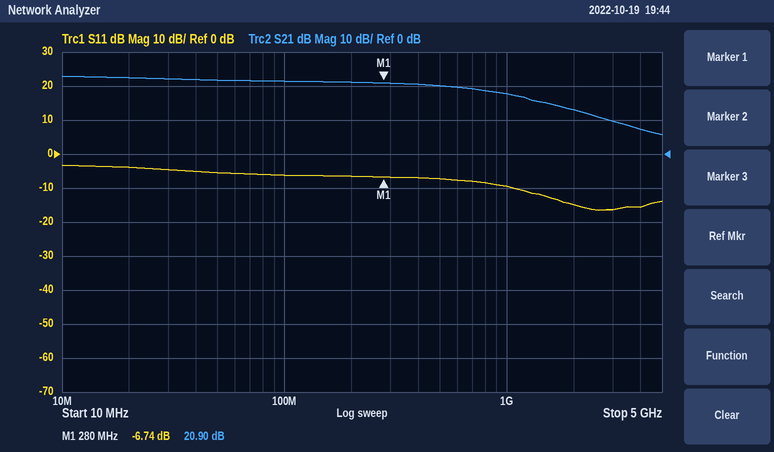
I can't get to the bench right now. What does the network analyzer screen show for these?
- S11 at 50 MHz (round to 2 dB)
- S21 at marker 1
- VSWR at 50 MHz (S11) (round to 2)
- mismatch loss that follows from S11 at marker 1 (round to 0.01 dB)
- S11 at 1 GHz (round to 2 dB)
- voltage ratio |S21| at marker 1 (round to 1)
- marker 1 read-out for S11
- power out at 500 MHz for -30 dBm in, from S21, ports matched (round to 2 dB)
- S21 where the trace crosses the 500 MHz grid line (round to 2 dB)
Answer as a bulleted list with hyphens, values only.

- -6 dB
- 20.90 dB
- 4
- 1.03 dB
- -10 dB
- 11
- -6.74 dB
- -10 dBm
- 20 dB
